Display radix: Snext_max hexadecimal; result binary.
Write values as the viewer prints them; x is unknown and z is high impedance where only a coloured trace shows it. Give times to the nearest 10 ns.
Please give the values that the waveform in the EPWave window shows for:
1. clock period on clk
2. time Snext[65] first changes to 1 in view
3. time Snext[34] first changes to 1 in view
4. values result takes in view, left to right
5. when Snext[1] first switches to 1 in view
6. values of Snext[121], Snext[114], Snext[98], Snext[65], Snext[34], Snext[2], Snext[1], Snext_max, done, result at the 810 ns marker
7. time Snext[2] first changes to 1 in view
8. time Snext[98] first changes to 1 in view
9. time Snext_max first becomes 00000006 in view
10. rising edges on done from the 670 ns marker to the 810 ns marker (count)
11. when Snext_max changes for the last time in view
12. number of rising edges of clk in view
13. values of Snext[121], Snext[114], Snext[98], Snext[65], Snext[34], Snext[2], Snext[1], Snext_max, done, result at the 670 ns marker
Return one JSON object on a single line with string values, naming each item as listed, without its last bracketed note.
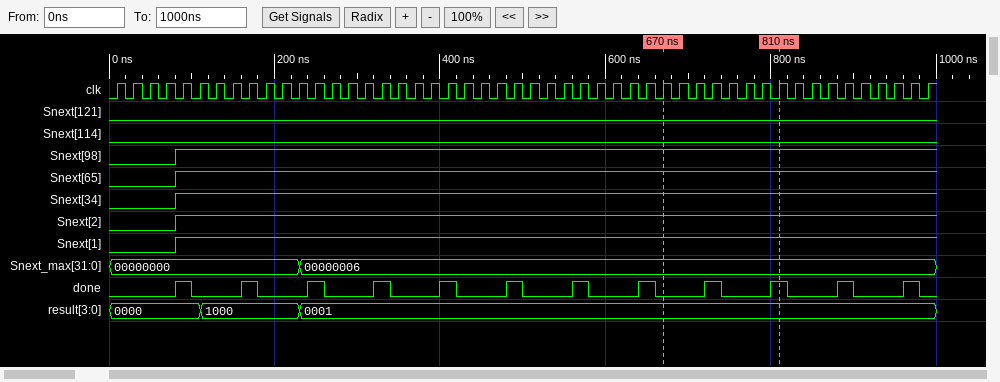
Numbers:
{"clock period on clk": "20 ns", "time Snext[65] first changes to 1 in view": "80 ns", "time Snext[34] first changes to 1 in view": "80 ns", "values result takes in view, left to right": "0000, 1000, 0001", "when Snext[1] first switches to 1 in view": "80 ns", "values of Snext[121], Snext[114], Snext[98], Snext[65], Snext[34], Snext[2], Snext[1], Snext_max, done, result at the 810 ns marker": "Snext[121]=0, Snext[114]=0, Snext[98]=1, Snext[65]=1, Snext[34]=1, Snext[2]=1, Snext[1]=1, Snext_max=00000006, done=1, result=0001", "time Snext[2] first changes to 1 in view": "80 ns", "time Snext[98] first changes to 1 in view": "80 ns", "time Snext_max first becomes 00000006 in view": "230 ns", "rising edges on done from the 670 ns marker to the 810 ns marker": "2", "when Snext_max changes for the last time in view": "230 ns", "number of rising edges of clk in view": "50", "values of Snext[121], Snext[114], Snext[98], Snext[65], Snext[34], Snext[2], Snext[1], Snext_max, done, result at the 670 ns marker": "Snext[121]=0, Snext[114]=0, Snext[98]=1, Snext[65]=1, Snext[34]=1, Snext[2]=1, Snext[1]=1, Snext_max=00000006, done=0, result=0001"}
